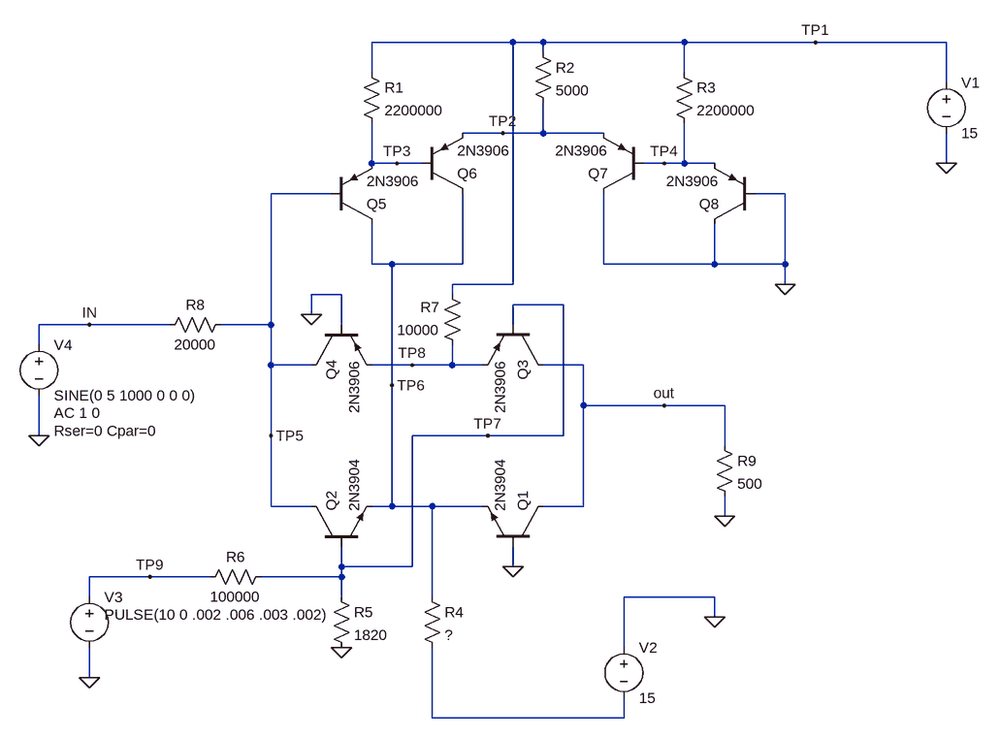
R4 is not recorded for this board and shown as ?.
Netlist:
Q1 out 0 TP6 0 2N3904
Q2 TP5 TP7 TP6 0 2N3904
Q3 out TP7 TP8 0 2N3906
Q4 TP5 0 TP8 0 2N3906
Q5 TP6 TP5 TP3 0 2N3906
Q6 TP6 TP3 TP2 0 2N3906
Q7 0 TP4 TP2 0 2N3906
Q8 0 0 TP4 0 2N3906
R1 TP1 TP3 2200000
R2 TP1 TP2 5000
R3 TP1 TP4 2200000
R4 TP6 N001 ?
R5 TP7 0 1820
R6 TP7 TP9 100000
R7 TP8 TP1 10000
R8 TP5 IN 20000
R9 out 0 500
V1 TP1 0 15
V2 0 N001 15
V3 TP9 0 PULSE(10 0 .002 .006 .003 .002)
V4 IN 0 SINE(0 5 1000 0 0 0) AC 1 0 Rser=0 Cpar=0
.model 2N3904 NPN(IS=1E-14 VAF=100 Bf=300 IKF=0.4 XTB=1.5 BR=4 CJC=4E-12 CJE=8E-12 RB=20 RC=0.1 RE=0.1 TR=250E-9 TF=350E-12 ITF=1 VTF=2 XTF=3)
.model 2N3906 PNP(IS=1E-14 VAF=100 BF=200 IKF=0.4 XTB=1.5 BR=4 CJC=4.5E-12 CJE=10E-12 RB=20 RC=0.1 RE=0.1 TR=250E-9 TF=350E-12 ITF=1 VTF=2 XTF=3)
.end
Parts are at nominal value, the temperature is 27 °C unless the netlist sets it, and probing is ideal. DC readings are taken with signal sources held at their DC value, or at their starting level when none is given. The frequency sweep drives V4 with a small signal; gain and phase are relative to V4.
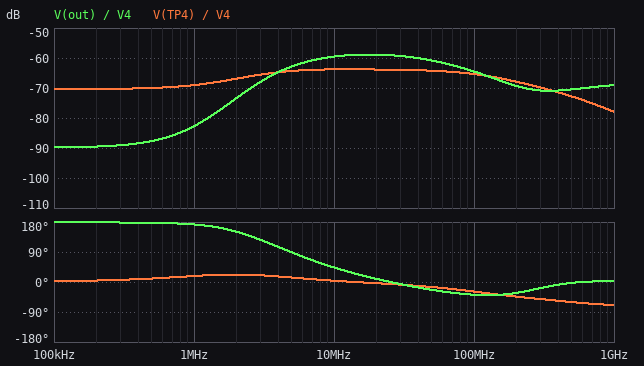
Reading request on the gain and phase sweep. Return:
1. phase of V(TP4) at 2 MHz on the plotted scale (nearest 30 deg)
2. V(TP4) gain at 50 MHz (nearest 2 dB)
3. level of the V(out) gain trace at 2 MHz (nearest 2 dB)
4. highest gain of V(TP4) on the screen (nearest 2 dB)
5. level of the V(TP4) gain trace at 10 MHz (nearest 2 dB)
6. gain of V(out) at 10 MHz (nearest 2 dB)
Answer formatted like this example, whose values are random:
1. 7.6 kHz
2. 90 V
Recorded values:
1. 30 deg
2. -64 dB
3. -74 dB
4. -64 dB
5. -64 dB
6. -60 dB
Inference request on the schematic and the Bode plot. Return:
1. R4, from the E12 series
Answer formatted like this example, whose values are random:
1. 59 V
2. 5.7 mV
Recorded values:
1. 10 kΩ
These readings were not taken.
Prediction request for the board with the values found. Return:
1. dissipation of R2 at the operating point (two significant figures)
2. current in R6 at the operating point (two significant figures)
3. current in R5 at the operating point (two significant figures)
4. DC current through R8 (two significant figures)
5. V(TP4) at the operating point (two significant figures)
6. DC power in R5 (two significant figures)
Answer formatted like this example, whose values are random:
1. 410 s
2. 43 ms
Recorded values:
1. 38 mW
2. 98 µA
3. 94 µA
4. 7.8 µA
5. 550 mV
6. 16 µW
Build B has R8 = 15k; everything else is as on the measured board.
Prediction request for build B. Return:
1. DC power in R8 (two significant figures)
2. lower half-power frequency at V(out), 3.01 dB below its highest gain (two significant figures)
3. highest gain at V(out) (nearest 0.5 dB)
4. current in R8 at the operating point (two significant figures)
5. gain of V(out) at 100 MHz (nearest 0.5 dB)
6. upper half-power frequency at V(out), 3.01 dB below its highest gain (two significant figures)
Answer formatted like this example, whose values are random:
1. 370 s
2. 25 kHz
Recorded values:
1. 1.6 µW
2. 6.1 MHz
3. -56.5 dB
4. 10 µA
5. -62.0 dB
6. 64 MHz
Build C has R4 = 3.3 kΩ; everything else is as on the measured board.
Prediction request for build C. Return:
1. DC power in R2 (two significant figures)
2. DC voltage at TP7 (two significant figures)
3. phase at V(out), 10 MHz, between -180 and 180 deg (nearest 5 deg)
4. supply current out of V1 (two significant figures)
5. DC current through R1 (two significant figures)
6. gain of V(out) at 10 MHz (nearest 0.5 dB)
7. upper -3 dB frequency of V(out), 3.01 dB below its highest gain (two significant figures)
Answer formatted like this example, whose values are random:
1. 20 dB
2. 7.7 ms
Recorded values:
1. 41 mW
2. 94 mV
3. -20 deg
4. 4.3 mA
5. 6.8 µA
6. -46.5 dB
7. 19 MHz
